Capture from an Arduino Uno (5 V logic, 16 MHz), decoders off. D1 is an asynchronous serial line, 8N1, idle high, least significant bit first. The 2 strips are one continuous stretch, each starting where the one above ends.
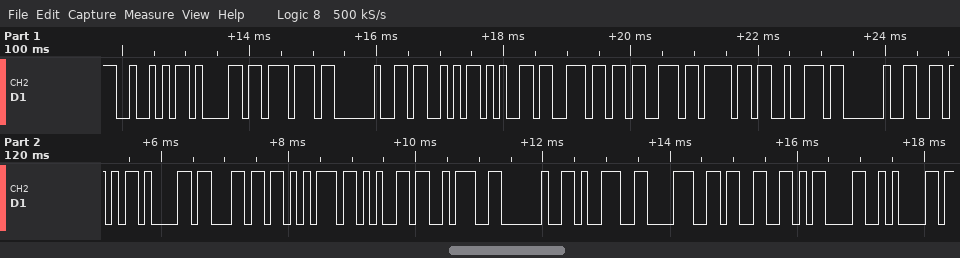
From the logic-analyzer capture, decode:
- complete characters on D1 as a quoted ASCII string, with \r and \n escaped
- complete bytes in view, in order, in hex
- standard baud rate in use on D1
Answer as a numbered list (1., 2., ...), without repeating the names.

1. "Raw Sensor Value: 983\r\n"
2. 52 61 77 20 53 65 6E 73 6F 72 20 56 61 6C 75 65 3A 20 39 38 33 0D 0A
3. 9600 baud
